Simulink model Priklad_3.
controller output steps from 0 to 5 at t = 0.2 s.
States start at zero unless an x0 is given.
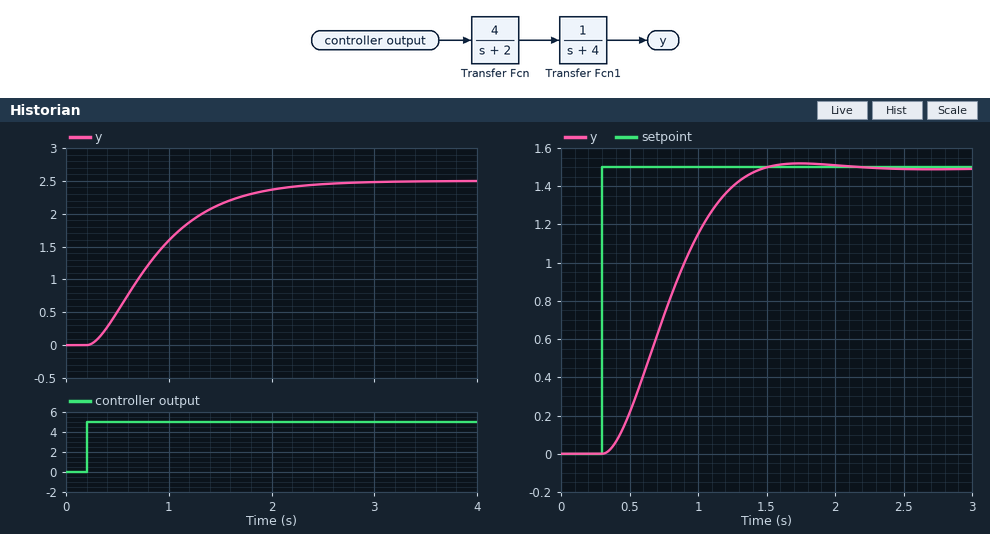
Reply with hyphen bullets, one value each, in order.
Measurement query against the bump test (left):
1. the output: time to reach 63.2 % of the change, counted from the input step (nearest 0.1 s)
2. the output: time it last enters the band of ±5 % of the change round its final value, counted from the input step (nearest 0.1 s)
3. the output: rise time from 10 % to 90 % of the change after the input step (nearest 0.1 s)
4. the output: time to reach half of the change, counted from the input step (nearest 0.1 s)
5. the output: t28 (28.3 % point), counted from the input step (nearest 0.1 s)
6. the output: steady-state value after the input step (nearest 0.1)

- 0.8 s
- 1.8 s
- 1.3 s
- 0.6 s
- 0.4 s
- 2.5
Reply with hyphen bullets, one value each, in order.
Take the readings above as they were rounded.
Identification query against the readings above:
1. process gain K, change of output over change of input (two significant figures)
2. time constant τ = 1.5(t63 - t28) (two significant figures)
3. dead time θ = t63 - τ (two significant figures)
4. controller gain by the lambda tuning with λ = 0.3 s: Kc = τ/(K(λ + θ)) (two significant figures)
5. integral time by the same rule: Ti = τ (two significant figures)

- 0.50
- 0.60 s
- 0.20 s
- 2.4
- 0.60 s
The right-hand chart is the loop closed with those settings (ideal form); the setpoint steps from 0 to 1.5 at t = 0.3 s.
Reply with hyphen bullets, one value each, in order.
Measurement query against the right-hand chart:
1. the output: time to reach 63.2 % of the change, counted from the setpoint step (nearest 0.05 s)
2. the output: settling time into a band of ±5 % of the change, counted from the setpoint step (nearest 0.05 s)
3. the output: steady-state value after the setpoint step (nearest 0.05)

- 0.55 s
- 1.00 s
- 1.50
